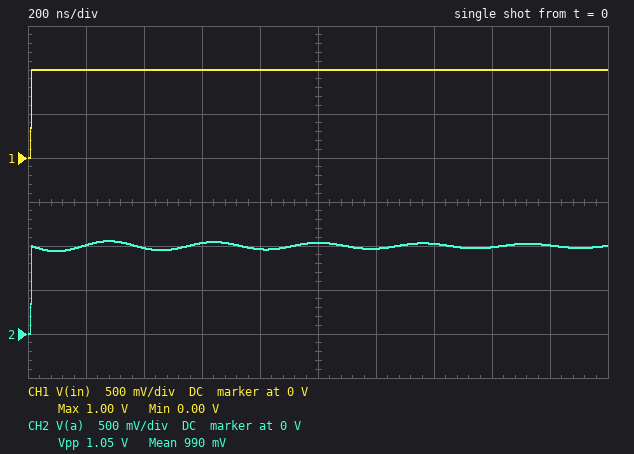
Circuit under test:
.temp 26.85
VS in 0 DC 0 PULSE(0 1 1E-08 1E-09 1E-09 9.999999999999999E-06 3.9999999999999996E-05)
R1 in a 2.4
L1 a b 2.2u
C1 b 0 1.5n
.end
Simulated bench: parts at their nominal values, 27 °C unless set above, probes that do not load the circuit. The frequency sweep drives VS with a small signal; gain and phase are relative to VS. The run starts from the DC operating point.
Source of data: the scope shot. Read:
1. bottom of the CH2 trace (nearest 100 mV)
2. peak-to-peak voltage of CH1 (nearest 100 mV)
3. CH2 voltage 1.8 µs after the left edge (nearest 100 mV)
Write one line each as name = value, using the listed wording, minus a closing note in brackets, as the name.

bottom of the CH2 trace = 0 V
peak-to-peak voltage of CH1 = 1.0 V
CH2 voltage 1.8 µs after the left edge = 1.0 V
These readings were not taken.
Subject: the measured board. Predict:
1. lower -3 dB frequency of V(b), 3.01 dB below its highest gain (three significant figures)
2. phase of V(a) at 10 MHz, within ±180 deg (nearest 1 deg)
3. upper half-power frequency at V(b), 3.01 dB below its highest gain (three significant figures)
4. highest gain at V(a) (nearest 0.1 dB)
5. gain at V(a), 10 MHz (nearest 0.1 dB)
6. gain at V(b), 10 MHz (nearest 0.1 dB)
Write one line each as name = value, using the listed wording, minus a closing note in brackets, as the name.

lower -3 dB frequency of V(b), 3.01 dB below its highest gain = 2.68 MHz
phase of V(a) at 10 MHz, within ±180 deg = 1 deg
upper half-power frequency at V(b), 3.01 dB below its highest gain = 2.85 MHz
highest gain at V(a) = 0 dB
gain at V(a), 10 MHz = 0 dB
gain at V(b), 10 MHz = -21.6 dB
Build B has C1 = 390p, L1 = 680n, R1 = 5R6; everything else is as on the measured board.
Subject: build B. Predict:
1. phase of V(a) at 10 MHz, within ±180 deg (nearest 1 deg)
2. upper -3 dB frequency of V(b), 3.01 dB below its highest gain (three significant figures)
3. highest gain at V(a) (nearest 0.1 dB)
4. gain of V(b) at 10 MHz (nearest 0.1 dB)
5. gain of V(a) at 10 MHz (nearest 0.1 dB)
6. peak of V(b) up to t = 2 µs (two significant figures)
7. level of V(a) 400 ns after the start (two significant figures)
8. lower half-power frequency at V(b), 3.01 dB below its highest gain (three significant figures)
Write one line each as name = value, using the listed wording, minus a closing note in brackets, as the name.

phase of V(a) at 10 MHz, within ±180 deg = 71 deg
upper -3 dB frequency of V(b), 3.01 dB below its highest gain = 10.4 MHz
highest gain at V(a) = 0 dB
gain of V(b) at 10 MHz = 16.8 dB
gain of V(a) at 10 MHz = -9.8 dB
peak of V(b) up to t = 2 µs = 1.8 V
level of V(a) 400 ns after the start = 1.0 V
lower half-power frequency at V(b), 3.01 dB below its highest gain = 9.05 MHz
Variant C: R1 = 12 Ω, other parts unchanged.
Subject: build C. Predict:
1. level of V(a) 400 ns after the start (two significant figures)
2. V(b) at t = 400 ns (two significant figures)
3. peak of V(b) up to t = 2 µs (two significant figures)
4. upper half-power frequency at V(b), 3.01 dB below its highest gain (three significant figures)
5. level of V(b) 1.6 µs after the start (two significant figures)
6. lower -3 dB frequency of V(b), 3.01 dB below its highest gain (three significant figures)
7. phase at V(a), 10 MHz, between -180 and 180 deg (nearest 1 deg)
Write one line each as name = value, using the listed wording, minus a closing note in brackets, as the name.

level of V(a) 400 ns after the start = 960 mV
V(b) at t = 400 ns = 660 mV
peak of V(b) up to t = 2 µs = 1.6 V
upper half-power frequency at V(b), 3.01 dB below its highest gain = 3.11 MHz
level of V(b) 1.6 µs after the start = 1.0 V
lower -3 dB frequency of V(b), 3.01 dB below its highest gain = 2.22 MHz
phase at V(a), 10 MHz, between -180 and 180 deg = 5 deg
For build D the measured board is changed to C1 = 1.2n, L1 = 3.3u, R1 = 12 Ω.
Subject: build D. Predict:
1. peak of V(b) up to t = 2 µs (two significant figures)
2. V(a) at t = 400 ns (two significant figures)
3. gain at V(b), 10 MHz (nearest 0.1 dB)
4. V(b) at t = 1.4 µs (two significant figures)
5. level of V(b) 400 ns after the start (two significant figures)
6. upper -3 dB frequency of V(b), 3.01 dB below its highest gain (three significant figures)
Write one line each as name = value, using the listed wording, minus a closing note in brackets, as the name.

peak of V(b) up to t = 2 µs = 1.7 V
V(a) at t = 400 ns = 1.0 V
gain at V(b), 10 MHz = -23.3 dB
V(b) at t = 1.4 µs = 1.1 V
level of V(b) 400 ns after the start = 520 mV
upper -3 dB frequency of V(b), 3.01 dB below its highest gain = 2.77 MHz
